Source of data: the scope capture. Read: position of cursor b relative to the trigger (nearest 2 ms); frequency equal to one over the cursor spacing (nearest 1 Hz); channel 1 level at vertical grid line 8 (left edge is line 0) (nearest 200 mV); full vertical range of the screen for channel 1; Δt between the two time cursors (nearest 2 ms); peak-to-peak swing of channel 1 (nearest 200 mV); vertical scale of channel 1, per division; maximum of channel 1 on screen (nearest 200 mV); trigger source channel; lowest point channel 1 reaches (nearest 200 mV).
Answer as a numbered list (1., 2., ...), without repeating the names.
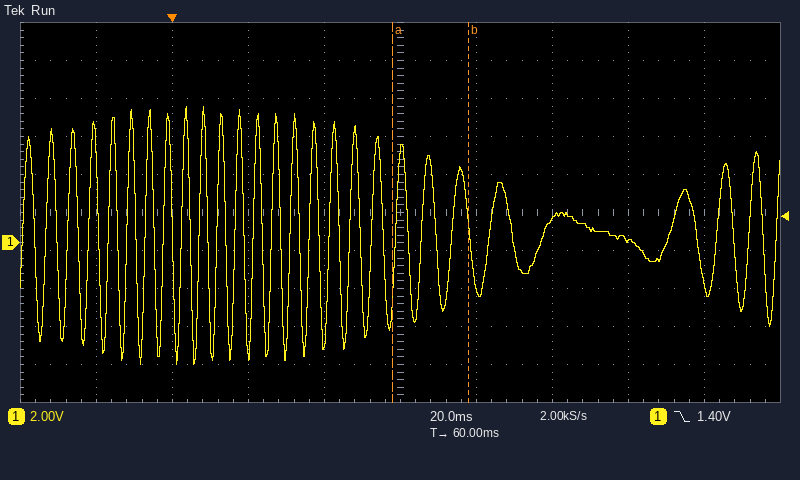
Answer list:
1. +78 ms
2. 50 Hz
3. 200 mV
4. 20 V
5. 20 ms
6. 13.6 V
7. 2 V
8. 7.2 V
9. channel 1
10. -6.4 V
